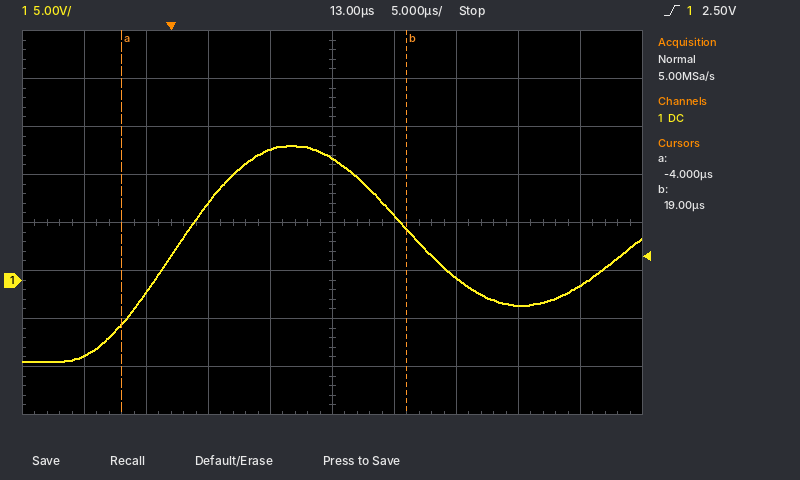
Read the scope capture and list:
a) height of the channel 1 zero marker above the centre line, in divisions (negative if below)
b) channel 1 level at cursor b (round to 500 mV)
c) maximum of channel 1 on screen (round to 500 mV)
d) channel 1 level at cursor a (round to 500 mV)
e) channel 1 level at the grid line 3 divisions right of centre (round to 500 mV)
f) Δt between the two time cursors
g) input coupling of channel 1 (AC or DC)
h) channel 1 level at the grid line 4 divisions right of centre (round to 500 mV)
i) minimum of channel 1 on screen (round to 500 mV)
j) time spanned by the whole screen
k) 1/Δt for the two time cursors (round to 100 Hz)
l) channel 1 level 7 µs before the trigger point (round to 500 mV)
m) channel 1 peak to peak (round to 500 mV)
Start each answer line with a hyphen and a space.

- -1.2 div
- 5.5 V
- 14.0 V
- -4.5 V
- -2.5 V
- 23.0 µs
- DC
- -500 mV
- -8.5 V
- 50 µs
- 43.5 kHz
- -8.0 V
- 22.5 V
